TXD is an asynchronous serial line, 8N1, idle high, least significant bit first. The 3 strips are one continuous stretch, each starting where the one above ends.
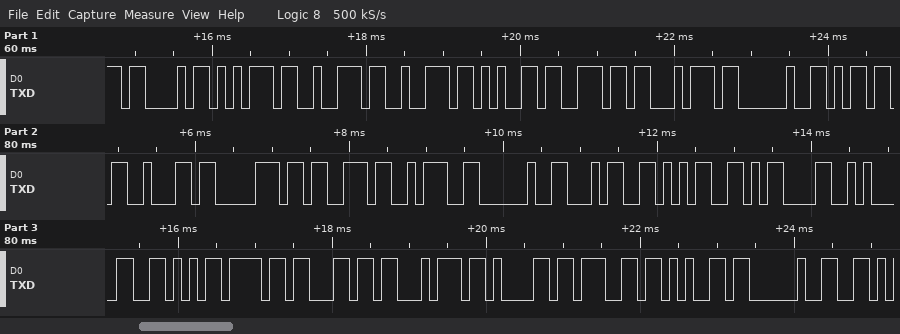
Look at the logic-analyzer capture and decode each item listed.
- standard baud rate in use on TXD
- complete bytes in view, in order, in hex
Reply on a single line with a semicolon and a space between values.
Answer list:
9600 baud; 43 75 72 72 65 6E 74 20 6D 62 70 73 3A 20 34 35 0D 0A 56 6F 6C 74 61 67 65 20
